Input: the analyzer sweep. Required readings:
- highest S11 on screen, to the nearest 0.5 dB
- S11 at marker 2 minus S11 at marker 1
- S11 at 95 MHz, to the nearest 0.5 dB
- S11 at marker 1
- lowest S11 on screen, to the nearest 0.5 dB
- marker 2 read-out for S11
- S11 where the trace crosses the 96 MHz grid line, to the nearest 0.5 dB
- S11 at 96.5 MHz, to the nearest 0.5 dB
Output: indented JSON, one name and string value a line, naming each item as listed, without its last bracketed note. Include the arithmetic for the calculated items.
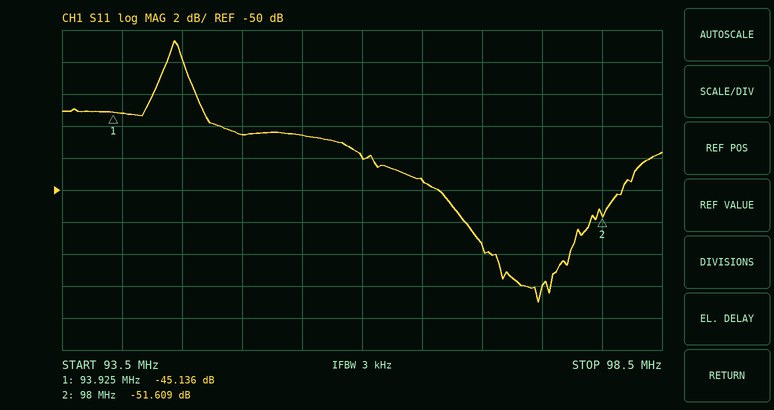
{
  "highest S11 on screen, to the nearest 0.5 dB": "-40.5 dB",
  "S11 at marker 2 minus S11 at marker 1": "-51.609 − (-45.136) = -6.473 dB",
  "S11 at 95 MHz, to the nearest 0.5 dB": "-46.5 dB",
  "S11 at marker 1": "-45.136 dB",
  "lowest S11 on screen, to the nearest 0.5 dB": "-57.0 dB",
  "marker 2 read-out for S11": "-51.609 dB",
  "S11 where the trace crosses the 96 MHz grid line, to the nearest 0.5 dB": "-48.0 dB",
  "S11 at 96.5 MHz, to the nearest 0.5 dB": "-49.5 dB"
}
